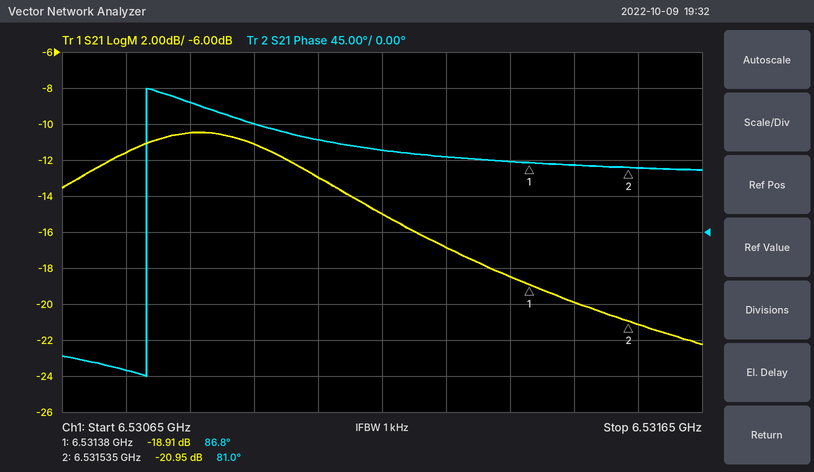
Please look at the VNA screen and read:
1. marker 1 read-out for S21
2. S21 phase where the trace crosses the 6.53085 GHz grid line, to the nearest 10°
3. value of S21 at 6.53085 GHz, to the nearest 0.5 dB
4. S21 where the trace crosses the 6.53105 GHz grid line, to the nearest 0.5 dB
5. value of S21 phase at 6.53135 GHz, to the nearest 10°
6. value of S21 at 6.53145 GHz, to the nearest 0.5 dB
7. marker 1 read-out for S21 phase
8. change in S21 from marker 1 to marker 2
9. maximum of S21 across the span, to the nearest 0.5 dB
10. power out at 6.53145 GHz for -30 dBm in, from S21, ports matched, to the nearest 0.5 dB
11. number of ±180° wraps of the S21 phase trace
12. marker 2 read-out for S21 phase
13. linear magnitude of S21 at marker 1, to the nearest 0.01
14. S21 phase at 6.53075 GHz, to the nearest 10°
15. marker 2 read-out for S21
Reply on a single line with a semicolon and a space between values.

-18.91 dB; 160°; -10.5 dB; -13.0 dB; 90°; -20.0 dB; 86.8°; -2.04 dB; -10.5 dB; -50.0 dBm; 1; 81.0°; 0.11; -170°; -20.95 dB
